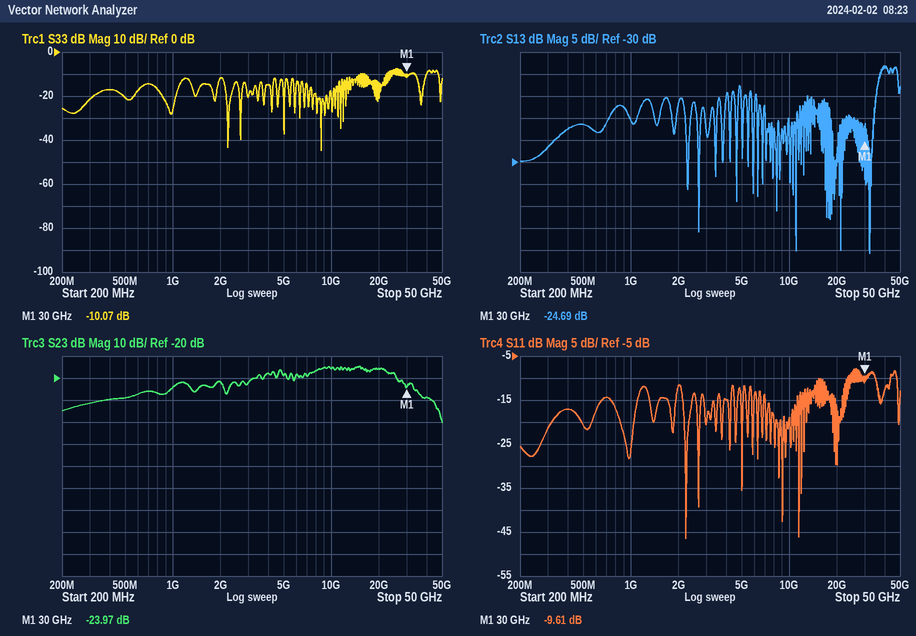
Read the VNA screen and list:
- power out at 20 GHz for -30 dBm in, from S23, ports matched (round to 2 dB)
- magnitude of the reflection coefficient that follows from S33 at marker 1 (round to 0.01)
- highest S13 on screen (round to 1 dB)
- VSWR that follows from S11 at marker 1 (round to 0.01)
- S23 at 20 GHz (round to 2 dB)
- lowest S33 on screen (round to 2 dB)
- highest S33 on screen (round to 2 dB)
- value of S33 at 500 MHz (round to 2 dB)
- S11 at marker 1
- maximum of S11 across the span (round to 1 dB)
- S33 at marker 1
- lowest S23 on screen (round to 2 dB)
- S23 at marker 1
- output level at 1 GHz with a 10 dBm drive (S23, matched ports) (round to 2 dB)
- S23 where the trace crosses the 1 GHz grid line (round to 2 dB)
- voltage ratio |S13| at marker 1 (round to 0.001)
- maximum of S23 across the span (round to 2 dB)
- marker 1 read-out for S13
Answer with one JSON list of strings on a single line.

["-46 dBm", "0.31", "-8 dB", "1.99", "-16 dB", "-44 dB", "-8 dB", "-20 dB", "-9.61 dB", "-8 dB", "-10.07 dB", "-40 dB", "-23.97 dB", "-14 dBm", "-24 dB", "0.058", "-14 dB", "-24.69 dB"]
